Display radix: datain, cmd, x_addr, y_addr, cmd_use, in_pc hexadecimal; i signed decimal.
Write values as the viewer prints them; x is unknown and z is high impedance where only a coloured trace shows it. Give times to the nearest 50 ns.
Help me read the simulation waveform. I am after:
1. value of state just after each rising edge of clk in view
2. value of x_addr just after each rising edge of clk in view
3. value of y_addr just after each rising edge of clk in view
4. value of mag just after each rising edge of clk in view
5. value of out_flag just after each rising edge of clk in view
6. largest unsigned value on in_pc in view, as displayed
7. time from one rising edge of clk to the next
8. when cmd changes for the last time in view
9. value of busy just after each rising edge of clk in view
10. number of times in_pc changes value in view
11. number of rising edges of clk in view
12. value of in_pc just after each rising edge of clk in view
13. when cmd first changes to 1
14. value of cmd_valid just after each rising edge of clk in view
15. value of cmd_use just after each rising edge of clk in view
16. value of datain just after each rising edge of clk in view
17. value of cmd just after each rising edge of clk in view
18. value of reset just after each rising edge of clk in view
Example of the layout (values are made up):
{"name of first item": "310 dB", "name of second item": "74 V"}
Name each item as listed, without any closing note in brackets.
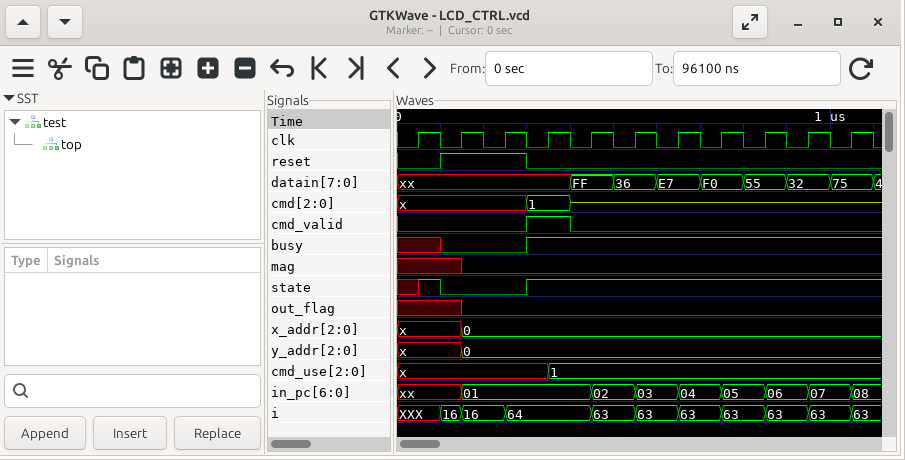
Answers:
{"value of state just after each rising edge of clk in view": "1 0 0 1 1 1 1 1 1 1 1", "value of x_addr just after each rising edge of clk in view": "x, 0, 0, 0, 0, 0, 0, 0, 0, 0, 0", "value of y_addr just after each rising edge of clk in view": "x, 0, 0, 0, 0, 0, 0, 0, 0, 0, 0", "value of mag just after each rising edge of clk in view": "x 0 0 0 0 0 0 0 0 0 0", "value of out_flag just after each rising edge of clk in view": "x 0 0 0 0 0 0 0 0 0 0", "largest unsigned value on in_pc in view, as displayed": "08", "time from one rising edge of clk to the next": "100 ns", "when cmd changes for the last time in view": "400 ns", "value of busy just after each rising edge of clk in view": "x 0 0 1 1 1 1 1 1 1 1", "number of times in_pc changes value in view": "8", "number of rising edges of clk in view": "11", "value of in_pc just after each rising edge of clk in view": "xx, 01, 01, 01, 02, 03, 04, 05, 06, 07, 08", "when cmd first changes to 1": "300 ns", "value of cmd_valid just after each rising edge of clk in view": "0 0 0 1 0 0 0 0 0 0 0", "value of cmd_use just after each rising edge of clk in view": "x, x, x, 1, 1, 1, 1, 1, 1, 1, 1", "value of datain just after each rising edge of clk in view": "xx, xx, xx, xx, FF, 36, E7, F0, 55, 32, 75", "value of cmd just after each rising edge of clk in view": "x, x, x, 1, z, z, z, z, z, z, z", "value of reset just after each rising edge of clk in view": "0 1 1 0 0 0 0 0 0 0 0"}
